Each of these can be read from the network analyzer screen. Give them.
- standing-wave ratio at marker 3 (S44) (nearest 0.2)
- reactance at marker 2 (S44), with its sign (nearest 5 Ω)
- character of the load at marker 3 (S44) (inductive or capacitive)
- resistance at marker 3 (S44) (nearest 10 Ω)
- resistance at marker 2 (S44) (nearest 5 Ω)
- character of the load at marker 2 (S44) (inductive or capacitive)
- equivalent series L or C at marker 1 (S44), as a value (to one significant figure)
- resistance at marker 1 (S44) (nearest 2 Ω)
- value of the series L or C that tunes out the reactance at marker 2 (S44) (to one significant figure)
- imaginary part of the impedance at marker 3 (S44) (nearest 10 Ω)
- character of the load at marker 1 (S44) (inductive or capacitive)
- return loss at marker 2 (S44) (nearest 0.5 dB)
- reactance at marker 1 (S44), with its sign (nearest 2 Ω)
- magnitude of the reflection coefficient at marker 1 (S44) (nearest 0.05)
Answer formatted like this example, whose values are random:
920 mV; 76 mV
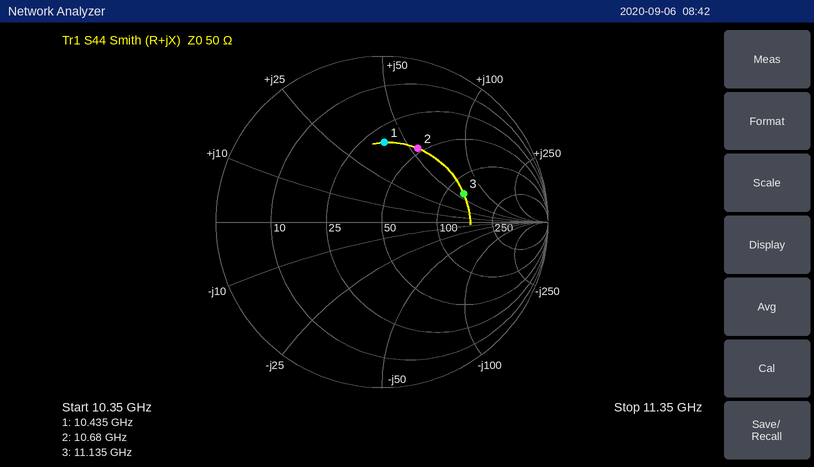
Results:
3.2; +55 Ω; inductive; 130 Ω; 45 Ω; inductive; 600 pH; 32 Ω; 300 fF; +60 Ω; inductive; 6.0 dB; +40 Ω; 0.50
